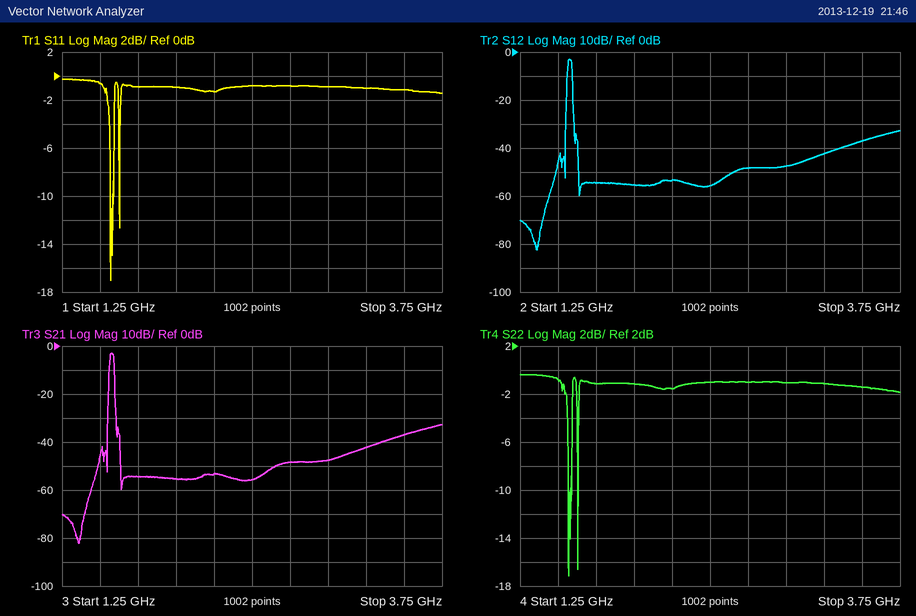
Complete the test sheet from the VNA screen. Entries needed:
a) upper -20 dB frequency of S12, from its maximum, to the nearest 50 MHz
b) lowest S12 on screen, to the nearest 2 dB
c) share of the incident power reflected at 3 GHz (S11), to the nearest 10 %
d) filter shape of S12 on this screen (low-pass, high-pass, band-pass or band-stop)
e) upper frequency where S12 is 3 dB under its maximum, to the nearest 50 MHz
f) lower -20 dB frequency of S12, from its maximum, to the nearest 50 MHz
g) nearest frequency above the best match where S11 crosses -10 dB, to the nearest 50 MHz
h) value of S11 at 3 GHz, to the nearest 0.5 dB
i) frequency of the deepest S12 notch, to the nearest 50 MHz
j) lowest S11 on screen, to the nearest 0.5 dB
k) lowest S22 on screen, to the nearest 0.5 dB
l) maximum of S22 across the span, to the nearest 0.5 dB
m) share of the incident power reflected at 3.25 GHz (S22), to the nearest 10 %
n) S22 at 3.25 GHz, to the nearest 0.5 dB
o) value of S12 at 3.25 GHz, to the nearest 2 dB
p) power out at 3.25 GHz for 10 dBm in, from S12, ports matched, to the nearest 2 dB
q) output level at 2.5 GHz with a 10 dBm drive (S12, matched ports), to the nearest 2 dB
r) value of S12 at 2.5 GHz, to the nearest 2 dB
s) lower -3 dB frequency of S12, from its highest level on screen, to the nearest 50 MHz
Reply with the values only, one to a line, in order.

1.60 GHz
-82 dB
80 %
band-pass
1.60 GHz
1.55 GHz
1.60 GHz
-1.0 dB
1.35 GHz
-17.0 dB
-17.0 dB
-0.5 dB
80 %
-1.0 dB
-42 dB
-32 dBm
-46 dBm
-56 dB
1.55 GHz
